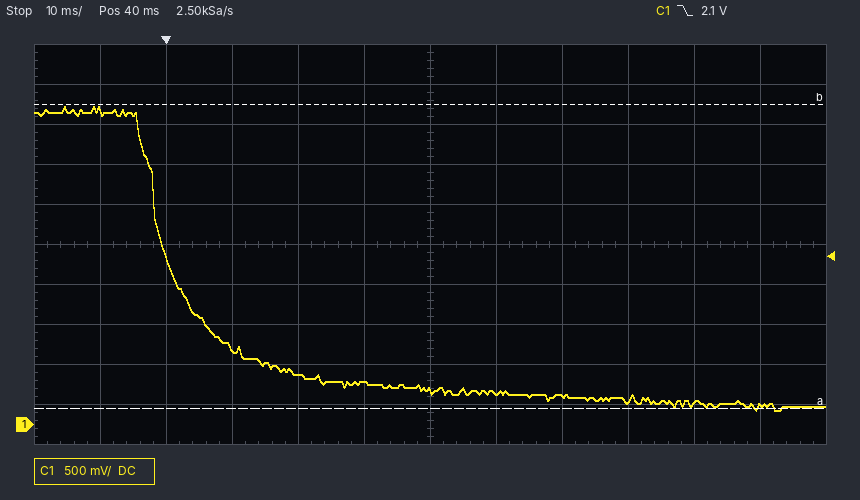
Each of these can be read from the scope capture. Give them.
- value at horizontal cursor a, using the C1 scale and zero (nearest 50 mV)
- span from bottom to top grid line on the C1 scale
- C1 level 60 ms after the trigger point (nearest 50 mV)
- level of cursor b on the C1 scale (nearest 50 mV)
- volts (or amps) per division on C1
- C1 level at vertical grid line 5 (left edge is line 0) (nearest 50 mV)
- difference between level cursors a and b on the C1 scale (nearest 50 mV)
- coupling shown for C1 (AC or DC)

200 mV
5 V
350 mV
4.00 V
500 mV
550 mV
3.80 V
DC
